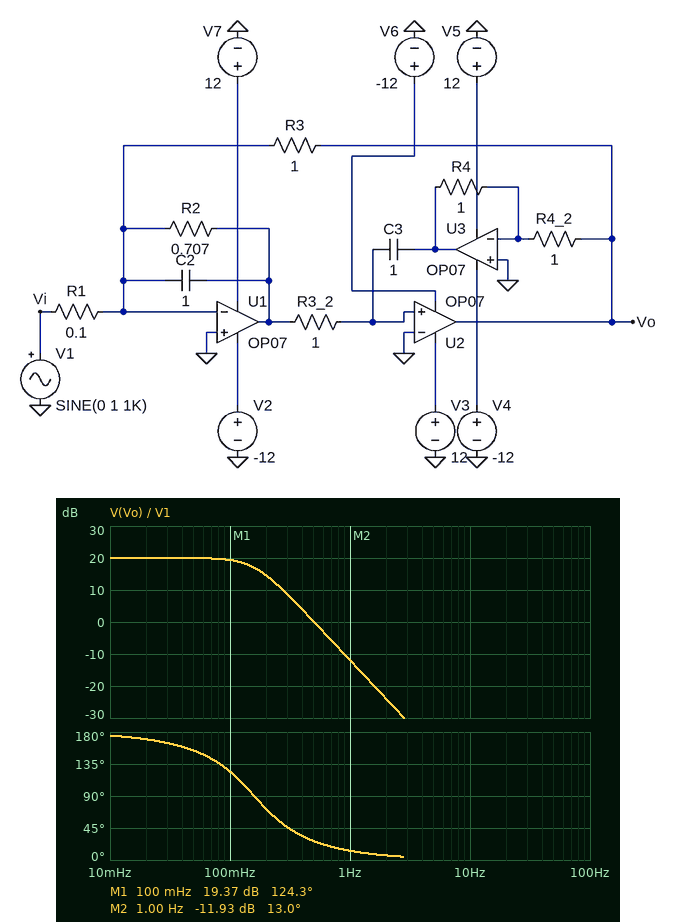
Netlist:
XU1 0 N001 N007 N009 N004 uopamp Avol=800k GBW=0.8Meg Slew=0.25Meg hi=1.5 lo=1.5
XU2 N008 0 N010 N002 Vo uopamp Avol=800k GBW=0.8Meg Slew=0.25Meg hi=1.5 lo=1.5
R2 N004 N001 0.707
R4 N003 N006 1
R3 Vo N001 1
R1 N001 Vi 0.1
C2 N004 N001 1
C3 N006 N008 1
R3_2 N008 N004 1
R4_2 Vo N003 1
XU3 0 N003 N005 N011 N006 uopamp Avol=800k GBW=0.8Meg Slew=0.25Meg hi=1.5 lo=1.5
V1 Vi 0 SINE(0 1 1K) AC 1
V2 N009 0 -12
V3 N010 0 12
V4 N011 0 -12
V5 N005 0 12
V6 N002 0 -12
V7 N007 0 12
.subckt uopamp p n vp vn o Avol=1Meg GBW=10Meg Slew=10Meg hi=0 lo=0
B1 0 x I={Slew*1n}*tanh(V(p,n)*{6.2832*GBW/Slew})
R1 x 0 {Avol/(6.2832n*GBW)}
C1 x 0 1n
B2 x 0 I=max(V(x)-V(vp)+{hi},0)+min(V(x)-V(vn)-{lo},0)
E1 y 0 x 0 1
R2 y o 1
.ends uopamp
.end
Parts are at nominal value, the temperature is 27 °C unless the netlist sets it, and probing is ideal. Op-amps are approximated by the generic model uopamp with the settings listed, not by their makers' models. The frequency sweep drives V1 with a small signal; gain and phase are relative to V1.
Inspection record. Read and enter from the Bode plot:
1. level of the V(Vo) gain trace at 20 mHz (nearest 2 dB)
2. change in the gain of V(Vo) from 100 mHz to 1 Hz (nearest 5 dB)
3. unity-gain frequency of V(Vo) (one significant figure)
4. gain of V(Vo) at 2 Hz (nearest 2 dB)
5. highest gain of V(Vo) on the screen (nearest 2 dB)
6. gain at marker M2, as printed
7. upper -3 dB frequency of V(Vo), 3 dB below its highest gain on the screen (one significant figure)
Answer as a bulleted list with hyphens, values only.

- 20 dB
- -30 dB
- 500 mHz
- -24 dB
- 20 dB
- -11.93 dB
- 200 mHz
